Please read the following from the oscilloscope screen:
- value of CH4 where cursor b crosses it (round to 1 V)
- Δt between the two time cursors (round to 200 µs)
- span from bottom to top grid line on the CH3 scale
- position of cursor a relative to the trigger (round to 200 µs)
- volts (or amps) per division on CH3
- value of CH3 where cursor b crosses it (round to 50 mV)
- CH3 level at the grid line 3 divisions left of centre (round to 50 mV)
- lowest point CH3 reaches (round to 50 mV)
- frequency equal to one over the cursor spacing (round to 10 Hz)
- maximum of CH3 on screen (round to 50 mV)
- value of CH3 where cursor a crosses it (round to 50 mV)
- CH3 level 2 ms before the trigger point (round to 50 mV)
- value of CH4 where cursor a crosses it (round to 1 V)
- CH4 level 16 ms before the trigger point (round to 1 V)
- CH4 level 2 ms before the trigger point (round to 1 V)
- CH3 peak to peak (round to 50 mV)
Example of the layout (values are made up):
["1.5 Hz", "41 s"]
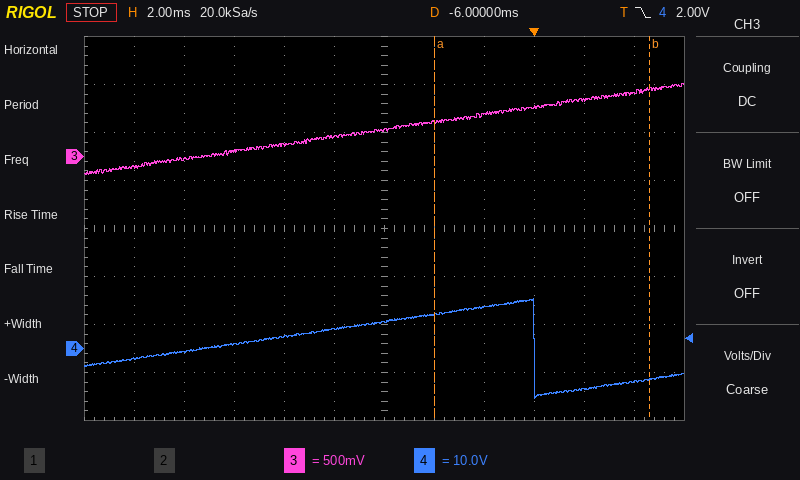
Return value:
["-6 V", "8.6 ms", "4 V", "-4.0 ms", "500 mV", "700 mV", "50 mV", "-200 mV", "120 Hz", "750 mV", "350 mV", "450 mV", "7 V", "-2 V", "9 V", "950 mV"]
